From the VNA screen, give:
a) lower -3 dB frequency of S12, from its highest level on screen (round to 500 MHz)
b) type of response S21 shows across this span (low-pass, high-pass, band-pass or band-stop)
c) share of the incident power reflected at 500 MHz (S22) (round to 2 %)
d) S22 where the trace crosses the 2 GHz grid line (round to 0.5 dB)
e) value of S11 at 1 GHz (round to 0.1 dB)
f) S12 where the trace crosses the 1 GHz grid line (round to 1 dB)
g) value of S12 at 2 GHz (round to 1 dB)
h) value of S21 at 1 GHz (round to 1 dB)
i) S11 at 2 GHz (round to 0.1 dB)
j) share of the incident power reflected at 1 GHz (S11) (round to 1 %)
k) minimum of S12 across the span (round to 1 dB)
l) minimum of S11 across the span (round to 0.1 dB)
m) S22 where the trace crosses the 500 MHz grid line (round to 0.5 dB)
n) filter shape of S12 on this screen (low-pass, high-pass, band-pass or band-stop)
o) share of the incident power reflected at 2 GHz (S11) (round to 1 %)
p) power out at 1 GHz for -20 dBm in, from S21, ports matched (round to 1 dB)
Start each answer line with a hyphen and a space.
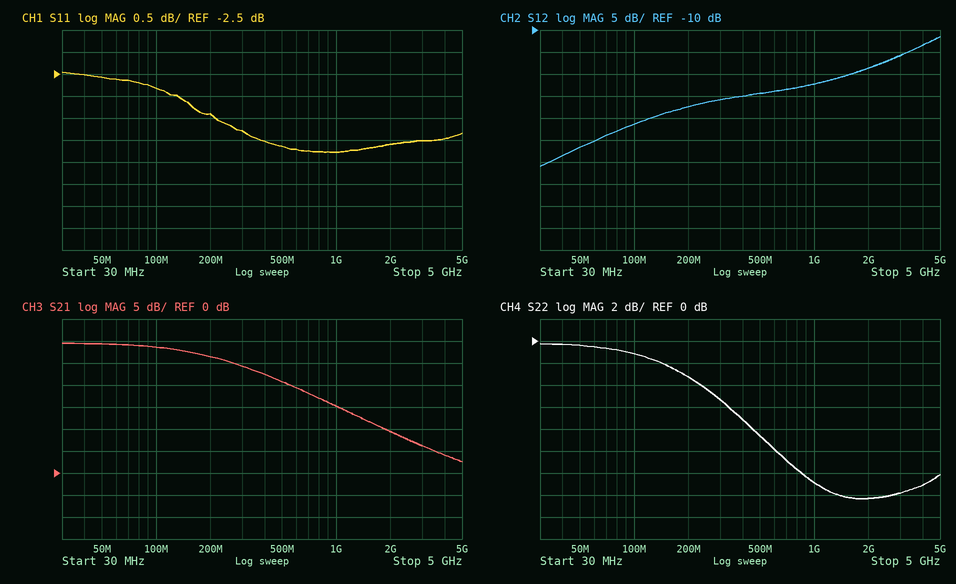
- 3.5 GHz
- low-pass
- 14 %
- -14.5 dB
- -4.3 dB
- -22 dB
- -19 dB
- 15 dB
- -4.1 dB
- 37 %
- -41 dB
- -4.3 dB
- -8.5 dB
- high-pass
- 39 %
- -5 dBm
